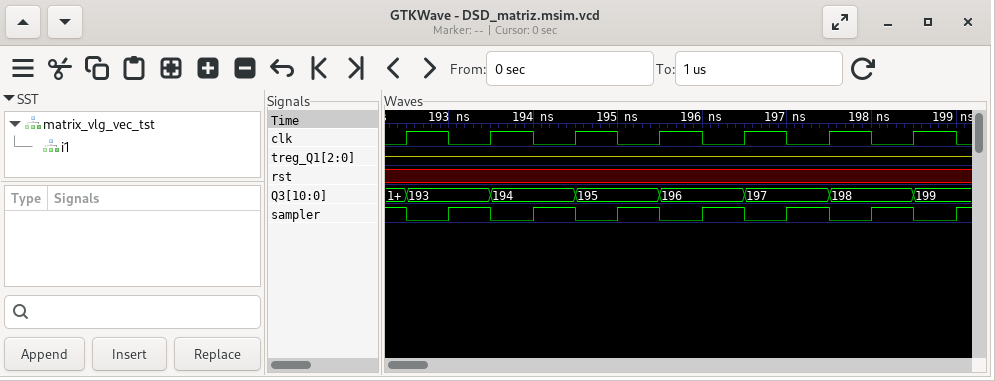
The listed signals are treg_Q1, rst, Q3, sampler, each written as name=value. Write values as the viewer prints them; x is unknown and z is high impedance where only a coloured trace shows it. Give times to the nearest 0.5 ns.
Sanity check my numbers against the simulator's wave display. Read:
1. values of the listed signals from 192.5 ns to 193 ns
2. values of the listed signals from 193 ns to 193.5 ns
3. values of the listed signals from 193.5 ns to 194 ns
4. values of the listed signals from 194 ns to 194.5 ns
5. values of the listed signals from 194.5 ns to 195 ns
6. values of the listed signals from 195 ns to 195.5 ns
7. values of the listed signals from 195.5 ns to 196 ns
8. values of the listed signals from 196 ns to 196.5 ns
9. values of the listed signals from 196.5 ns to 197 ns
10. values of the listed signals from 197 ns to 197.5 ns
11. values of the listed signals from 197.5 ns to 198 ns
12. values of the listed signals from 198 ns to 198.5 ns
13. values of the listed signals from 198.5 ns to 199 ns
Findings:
treg_Q1=z, rst=x, Q3=193, sampler=0
treg_Q1=z, rst=x, Q3=193, sampler=1
treg_Q1=z, rst=x, Q3=194, sampler=0
treg_Q1=z, rst=x, Q3=194, sampler=1
treg_Q1=z, rst=x, Q3=195, sampler=0
treg_Q1=z, rst=x, Q3=195, sampler=1
treg_Q1=z, rst=x, Q3=196, sampler=0
treg_Q1=z, rst=x, Q3=196, sampler=1
treg_Q1=z, rst=x, Q3=197, sampler=0
treg_Q1=z, rst=x, Q3=197, sampler=1
treg_Q1=z, rst=x, Q3=198, sampler=0
treg_Q1=z, rst=x, Q3=198, sampler=1
treg_Q1=z, rst=x, Q3=199, sampler=0
